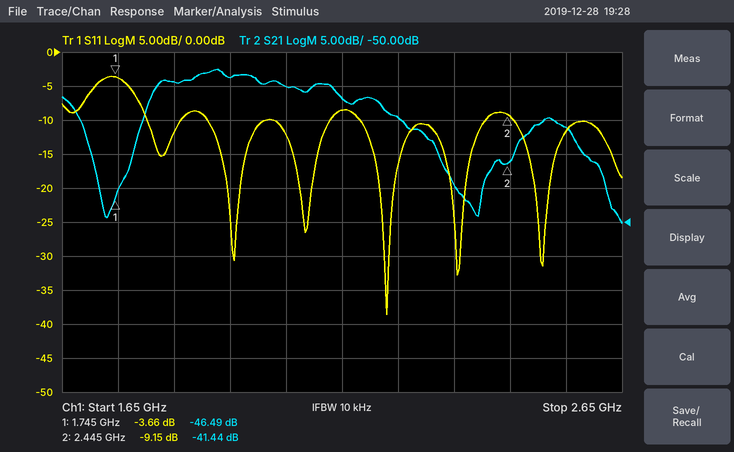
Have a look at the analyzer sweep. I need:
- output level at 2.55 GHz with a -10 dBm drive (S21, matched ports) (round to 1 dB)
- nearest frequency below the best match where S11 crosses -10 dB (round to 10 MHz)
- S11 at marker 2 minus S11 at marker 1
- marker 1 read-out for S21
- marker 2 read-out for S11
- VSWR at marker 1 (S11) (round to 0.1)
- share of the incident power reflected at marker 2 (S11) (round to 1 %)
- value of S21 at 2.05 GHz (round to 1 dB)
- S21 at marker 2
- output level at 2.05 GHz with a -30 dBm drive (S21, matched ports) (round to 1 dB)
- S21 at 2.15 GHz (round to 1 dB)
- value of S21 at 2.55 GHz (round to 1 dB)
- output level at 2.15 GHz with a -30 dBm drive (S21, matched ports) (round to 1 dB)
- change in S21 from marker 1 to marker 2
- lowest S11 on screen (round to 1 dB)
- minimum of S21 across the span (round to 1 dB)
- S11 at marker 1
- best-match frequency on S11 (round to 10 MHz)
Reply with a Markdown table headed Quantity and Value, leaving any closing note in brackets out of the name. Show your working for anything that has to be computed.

| Quantity | Value |
|---|---|
| output level at 2.55 GHz with a -10 dBm drive (S21, matched ports) | -10 dBm + (-36 dB) = -46 dBm |
| nearest frequency below the best match where S11 crosses -10 dB | 2.18 GHz |
| S11 at marker 2 minus S11 at marker 1 | -9.15 − (-3.66) = -5.49 dB |
| marker 1 read-out for S21 | -46.49 dB |
| marker 2 read-out for S11 | -9.15 dB |
| VSWR at marker 1 (S11) | (1 + 0.6561)/(1 − 0.6561) ≈ 4.8 |
| share of the incident power reflected at marker 2 (S11) | 10^(-9.15/10) ≈ 12 % |
| value of S21 at 2.05 GHz | -30 dB |
| S21 at marker 2 | -41.44 dB |
| output level at 2.05 GHz with a -30 dBm drive (S21, matched ports) | -30 dBm + (-30 dB) = -60 dBm |
| S21 at 2.15 GHz | -32 dB |
| value of S21 at 2.55 GHz | -36 dB |
| output level at 2.15 GHz with a -30 dBm drive (S21, matched ports) | -30 dBm + (-32 dB) = -62 dBm |
| change in S21 from marker 1 to marker 2 | -41.44 − (-46.49) = 5.05 dB |
| lowest S11 on screen | -39 dB |
| minimum of S21 across the span | -50 dB |
| S11 at marker 1 | -3.66 dB |
| best-match frequency on S11 | 2.23 GHz |
